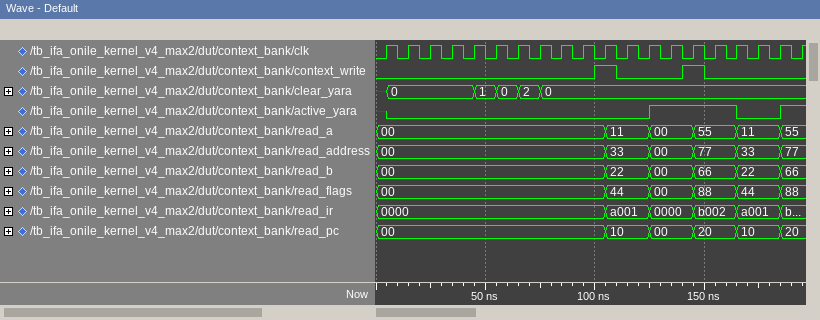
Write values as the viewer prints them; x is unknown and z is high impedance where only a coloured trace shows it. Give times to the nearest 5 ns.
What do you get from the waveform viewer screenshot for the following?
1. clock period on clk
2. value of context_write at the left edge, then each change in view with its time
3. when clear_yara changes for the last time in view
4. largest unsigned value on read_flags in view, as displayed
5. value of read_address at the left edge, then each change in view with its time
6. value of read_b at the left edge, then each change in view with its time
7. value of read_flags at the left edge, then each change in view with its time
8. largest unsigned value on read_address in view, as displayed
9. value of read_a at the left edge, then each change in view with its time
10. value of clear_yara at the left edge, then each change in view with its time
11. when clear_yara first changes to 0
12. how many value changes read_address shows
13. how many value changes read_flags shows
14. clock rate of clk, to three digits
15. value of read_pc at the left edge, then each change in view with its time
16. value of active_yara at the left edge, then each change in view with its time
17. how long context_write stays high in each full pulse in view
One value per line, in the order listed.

10 ns
0, 1 at 100 ns, 0 at 110 ns, 1 at 140 ns, 0 at 150 ns
75 ns
88
00, 33 at 105 ns, 00 at 125 ns, 77 at 145 ns, 33 at 165 ns, 77 at 185 ns
00, 22 at 105 ns, 00 at 125 ns, 66 at 145 ns, 22 at 165 ns, 66 at 185 ns
00, 44 at 105 ns, 00 at 125 ns, 88 at 145 ns, 44 at 165 ns, 88 at 185 ns
77
00, 11 at 105 ns, 00 at 125 ns, 55 at 145 ns, 11 at 165 ns, 55 at 185 ns
x, 0 at 5 ns, 1 at 45 ns, 0 at 55 ns, 2 at 65 ns, 0 at 75 ns
5 ns
5
5
100 MHz
00, 10 at 105 ns, 00 at 125 ns, 20 at 145 ns, 10 at 165 ns, 20 at 185 ns
x, 0 at 5 ns, 1 at 125 ns, 0 at 165 ns, 1 at 185 ns
10 ns, 10 ns
